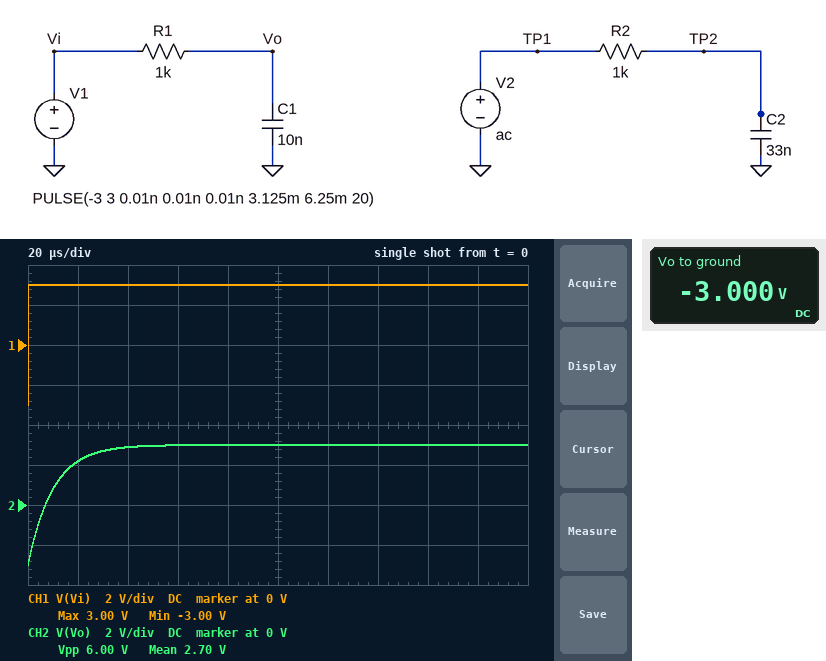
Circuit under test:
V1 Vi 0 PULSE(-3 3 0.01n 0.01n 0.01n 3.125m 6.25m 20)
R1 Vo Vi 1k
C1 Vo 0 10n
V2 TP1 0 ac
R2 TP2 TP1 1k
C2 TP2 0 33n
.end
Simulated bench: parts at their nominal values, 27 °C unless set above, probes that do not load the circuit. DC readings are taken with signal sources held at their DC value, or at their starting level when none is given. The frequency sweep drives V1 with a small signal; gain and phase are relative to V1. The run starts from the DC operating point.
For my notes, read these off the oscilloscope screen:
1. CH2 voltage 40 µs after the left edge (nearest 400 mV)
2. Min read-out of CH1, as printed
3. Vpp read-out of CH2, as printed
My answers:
2.8 V
-3.00 V
6.00 V
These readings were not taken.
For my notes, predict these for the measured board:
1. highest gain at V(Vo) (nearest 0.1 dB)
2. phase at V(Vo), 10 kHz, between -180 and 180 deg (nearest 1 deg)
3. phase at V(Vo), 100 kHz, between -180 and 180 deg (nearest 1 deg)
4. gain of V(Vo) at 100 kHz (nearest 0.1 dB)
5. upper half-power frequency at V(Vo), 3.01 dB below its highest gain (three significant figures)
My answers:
0 dB
-32 deg
-81 deg
-16.1 dB
15.9 kHz
